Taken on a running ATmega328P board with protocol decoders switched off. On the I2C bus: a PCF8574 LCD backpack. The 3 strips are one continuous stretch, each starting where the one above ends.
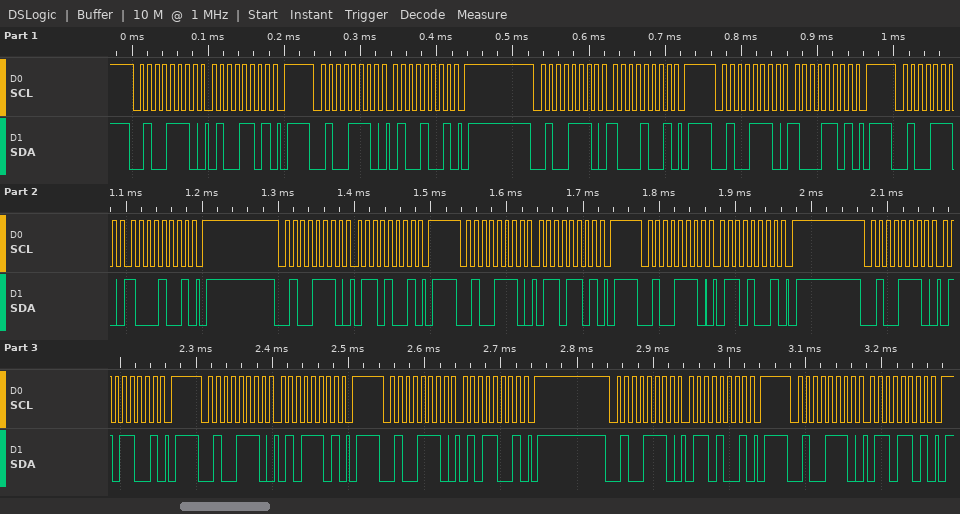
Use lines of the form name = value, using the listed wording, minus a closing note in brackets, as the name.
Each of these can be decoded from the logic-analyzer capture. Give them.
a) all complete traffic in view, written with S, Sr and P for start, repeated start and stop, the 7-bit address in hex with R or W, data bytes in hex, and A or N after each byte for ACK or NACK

all complete traffic in view, written with S, Sr and P for start, repeated start and stop, the 7-bit address in hex with R or W, data bytes in hex, and A or N after each byte for ACK or NACK = S 27W A 4D A P S 27W A 49 A P S 27W A 89 A P S 27W A 8D A P S 27W A 89 A P S 27W A 69 A P S 27W A 6D A P S 27W A 69 A P S 27W A 59 A P S 27W A 5D A P S 27W A 59 A P S 27W A 69 A P S 27W A 6D A P
